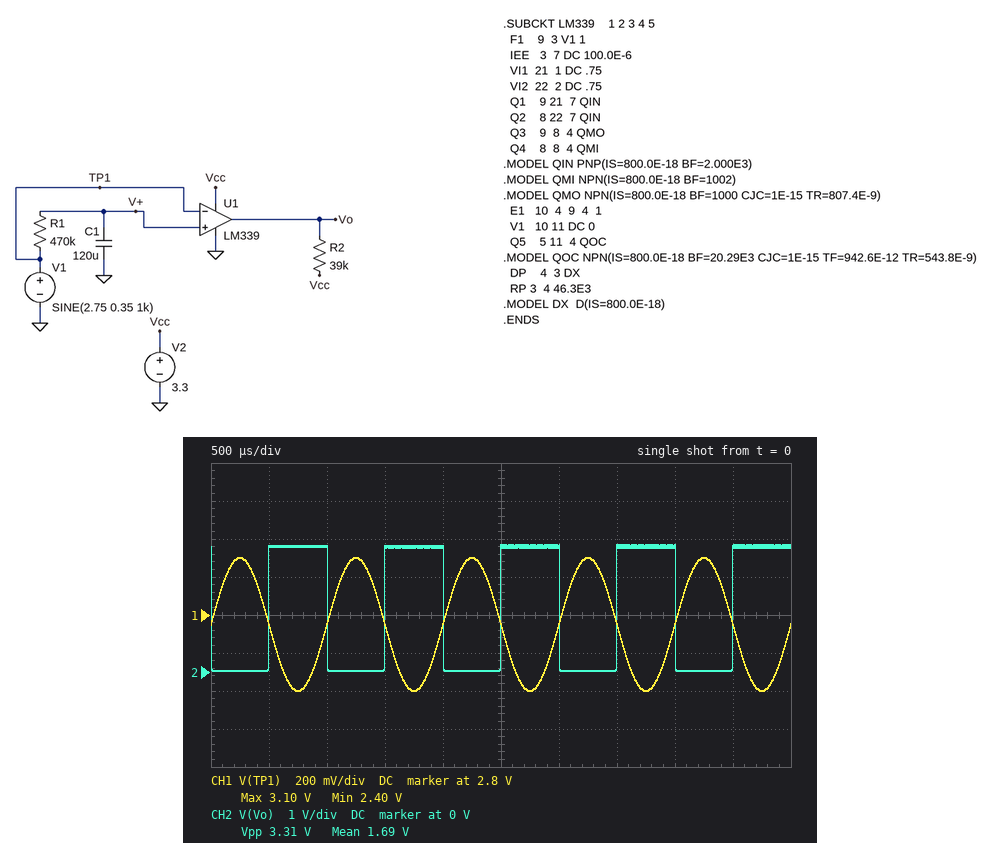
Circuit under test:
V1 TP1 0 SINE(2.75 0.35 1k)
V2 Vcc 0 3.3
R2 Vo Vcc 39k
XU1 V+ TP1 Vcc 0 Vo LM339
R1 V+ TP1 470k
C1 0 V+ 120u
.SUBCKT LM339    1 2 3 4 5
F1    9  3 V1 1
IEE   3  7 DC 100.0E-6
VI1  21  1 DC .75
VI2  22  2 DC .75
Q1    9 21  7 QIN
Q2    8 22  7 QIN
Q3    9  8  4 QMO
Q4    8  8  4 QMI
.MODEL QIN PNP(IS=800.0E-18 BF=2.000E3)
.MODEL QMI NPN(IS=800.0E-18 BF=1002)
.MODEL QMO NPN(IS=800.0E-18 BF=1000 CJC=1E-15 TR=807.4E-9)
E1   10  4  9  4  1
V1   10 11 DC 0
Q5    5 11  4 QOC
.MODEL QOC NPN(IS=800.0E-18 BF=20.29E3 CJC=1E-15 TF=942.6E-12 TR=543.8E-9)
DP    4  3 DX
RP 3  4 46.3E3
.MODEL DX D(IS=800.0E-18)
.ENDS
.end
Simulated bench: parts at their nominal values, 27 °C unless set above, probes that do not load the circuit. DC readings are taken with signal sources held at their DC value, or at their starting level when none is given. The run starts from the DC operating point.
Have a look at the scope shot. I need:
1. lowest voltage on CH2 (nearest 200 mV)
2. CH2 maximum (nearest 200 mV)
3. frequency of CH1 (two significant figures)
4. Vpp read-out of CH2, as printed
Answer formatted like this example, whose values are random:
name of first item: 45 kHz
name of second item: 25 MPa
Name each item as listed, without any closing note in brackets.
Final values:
lowest voltage on CH2: 0 V
CH2 maximum: 3.4 V
frequency of CH1: 1.0 kHz
Vpp read-out of CH2, as printed: 3.31 V
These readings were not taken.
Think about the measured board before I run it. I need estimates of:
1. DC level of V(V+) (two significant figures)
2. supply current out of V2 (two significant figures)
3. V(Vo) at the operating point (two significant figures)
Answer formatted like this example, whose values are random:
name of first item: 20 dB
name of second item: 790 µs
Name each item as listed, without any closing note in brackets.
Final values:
DC level of V(V+): 2.8 V
supply current out of V2: 170 µA
V(Vo) at the operating point: 3.3 V
